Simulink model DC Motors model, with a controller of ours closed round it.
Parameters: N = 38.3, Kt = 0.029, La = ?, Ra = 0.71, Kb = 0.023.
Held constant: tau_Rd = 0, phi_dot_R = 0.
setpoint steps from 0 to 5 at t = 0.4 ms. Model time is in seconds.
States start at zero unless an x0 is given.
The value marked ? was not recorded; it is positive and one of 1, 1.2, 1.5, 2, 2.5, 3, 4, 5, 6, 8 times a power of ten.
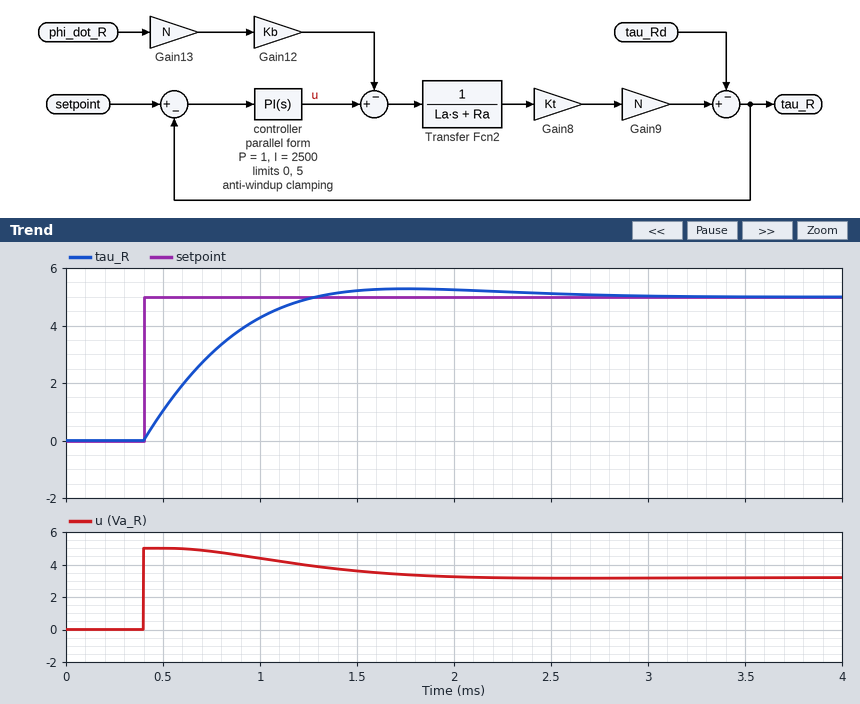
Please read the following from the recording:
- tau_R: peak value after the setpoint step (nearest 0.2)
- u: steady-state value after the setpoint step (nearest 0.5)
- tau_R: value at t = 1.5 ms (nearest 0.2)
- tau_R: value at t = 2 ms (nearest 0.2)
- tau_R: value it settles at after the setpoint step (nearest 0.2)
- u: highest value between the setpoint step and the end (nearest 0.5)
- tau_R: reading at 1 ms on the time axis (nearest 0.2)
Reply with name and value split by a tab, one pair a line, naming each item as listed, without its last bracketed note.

tau_R: peak value after the setpoint step	5.2
u: steady-state value after the setpoint step	3.0
tau_R: value at t = 1.5 ms	5.2
tau_R: value at t = 2 ms	5.2
tau_R: value it settles at after the setpoint step	5.0
u: highest value between the setpoint step and the end	5.0
tau_R: reading at 1 ms on the time axis	4.2
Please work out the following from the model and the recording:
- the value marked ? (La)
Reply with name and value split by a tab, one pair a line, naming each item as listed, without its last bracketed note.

the value marked ?	0.0005
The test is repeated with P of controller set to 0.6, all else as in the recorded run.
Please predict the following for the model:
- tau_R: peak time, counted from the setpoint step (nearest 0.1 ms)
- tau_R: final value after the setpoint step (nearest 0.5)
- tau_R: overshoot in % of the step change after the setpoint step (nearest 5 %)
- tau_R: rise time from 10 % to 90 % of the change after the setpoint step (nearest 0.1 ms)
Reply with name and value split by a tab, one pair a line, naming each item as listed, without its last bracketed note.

tau_R: peak time, counted from the setpoint step	1.3 ms
tau_R: final value after the setpoint step	5.0
tau_R: overshoot in % of the step change after the setpoint step	15 %
tau_R: rise time from 10 % to 90 % of the change after the setpoint step	0.6 ms
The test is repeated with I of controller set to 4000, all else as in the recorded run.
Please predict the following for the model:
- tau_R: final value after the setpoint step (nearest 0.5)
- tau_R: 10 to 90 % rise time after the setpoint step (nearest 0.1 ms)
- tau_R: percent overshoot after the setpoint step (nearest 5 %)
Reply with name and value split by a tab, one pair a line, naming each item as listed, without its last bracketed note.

tau_R: final value after the setpoint step	5.0
tau_R: 10 to 90 % rise time after the setpoint step	0.6 ms
tau_R: percent overshoot after the setpoint step	10 %
